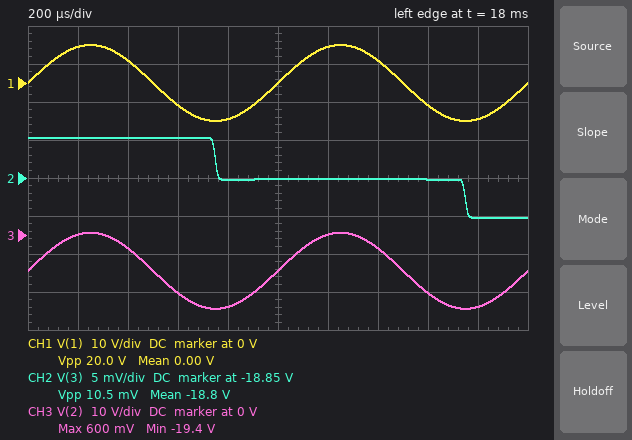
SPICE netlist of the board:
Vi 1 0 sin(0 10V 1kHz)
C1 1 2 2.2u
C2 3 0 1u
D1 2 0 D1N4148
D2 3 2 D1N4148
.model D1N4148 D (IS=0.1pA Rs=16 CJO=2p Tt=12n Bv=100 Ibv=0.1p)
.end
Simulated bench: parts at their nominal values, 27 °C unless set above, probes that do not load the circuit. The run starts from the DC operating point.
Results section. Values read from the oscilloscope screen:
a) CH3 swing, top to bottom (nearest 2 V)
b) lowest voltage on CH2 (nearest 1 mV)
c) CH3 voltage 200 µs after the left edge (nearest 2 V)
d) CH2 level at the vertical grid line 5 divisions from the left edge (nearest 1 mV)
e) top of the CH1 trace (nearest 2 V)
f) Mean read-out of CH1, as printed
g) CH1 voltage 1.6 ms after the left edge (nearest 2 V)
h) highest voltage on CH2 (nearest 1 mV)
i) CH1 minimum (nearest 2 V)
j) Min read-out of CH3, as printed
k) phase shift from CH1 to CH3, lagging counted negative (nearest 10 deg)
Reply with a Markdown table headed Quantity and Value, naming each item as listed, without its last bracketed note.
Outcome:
| Quantity | Value |
|---|---|
| CH3 swing, top to bottom | 20 V |
| lowest voltage on CH2 | -18.855 V |
| CH3 voltage 200 µs after the left edge | 0 V |
| CH2 level at the vertical grid line 5 divisions from the left edge | -18.850 V |
| top of the CH1 trace | 10 V |
| Mean read-out of CH1, as printed | 0.00 V |
| CH1 voltage 1.6 ms after the left edge | -6 V |
| highest voltage on CH2 | -18.845 V |
| CH1 minimum | -10 V |
| Min read-out of CH3, as printed | -19.4 V |
| phase shift from CH1 to CH3, lagging counted negative | 0 deg |
